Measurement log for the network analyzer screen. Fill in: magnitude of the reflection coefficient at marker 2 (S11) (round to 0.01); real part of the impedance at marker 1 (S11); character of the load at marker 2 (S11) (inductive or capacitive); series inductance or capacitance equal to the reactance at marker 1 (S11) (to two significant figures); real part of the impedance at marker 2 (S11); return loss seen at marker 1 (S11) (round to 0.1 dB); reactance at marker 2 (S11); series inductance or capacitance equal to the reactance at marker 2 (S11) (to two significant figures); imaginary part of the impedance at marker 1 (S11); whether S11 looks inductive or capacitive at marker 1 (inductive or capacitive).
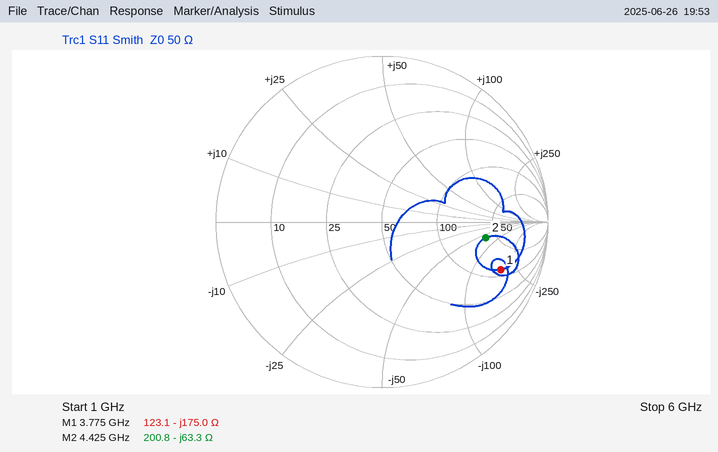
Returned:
0.63
123.1 Ω
capacitive
240 fF
200.8 Ω
2.3 dB
-63.3 Ω
570 fF
-175.0 Ω
capacitive
